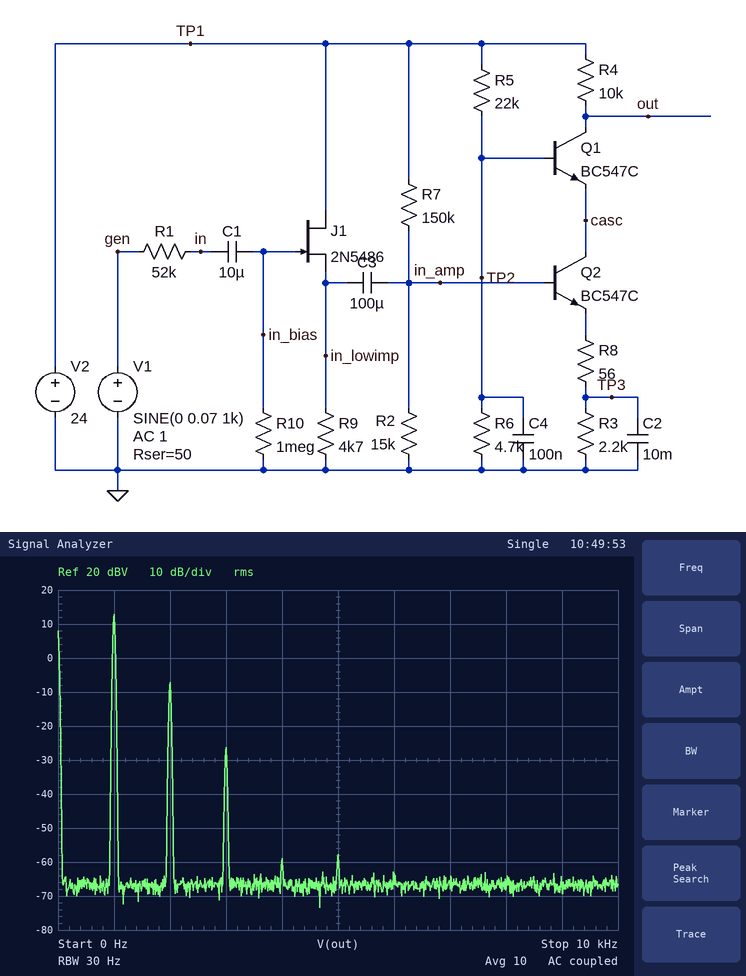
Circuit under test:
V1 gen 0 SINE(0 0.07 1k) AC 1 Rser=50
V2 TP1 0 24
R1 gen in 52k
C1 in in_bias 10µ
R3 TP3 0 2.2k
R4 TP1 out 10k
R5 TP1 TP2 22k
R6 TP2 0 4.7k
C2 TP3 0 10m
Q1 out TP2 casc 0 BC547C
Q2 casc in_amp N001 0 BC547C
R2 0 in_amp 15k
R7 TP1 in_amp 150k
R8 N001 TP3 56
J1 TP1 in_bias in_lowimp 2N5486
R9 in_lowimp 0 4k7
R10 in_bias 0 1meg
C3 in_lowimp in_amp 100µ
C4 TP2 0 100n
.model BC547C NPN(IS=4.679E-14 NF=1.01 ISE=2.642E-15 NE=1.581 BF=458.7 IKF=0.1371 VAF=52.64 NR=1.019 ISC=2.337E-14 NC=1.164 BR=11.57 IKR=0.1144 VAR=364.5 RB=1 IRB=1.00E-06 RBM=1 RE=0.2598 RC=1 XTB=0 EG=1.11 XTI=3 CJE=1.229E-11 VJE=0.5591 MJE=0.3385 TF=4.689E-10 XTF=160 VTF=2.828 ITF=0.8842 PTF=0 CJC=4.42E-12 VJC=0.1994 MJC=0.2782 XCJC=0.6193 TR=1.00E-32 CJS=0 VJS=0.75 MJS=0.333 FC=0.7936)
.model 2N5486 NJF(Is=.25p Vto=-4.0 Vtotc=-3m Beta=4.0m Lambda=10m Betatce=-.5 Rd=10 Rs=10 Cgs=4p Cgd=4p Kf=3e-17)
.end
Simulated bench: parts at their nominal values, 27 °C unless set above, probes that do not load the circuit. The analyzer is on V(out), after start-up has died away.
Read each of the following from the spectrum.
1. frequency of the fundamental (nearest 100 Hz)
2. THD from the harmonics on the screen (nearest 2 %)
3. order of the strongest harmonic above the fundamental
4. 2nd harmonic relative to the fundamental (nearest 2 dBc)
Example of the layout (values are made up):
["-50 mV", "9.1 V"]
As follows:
["1.0 kHz", "10 %", "2", "-20 dBc"]
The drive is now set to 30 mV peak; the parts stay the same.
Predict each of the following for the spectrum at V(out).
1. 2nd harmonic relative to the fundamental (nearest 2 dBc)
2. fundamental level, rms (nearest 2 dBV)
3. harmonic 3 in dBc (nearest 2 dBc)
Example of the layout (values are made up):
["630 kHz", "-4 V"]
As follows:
["-28 dBc", "6 dBV", "-54 dBc"]
